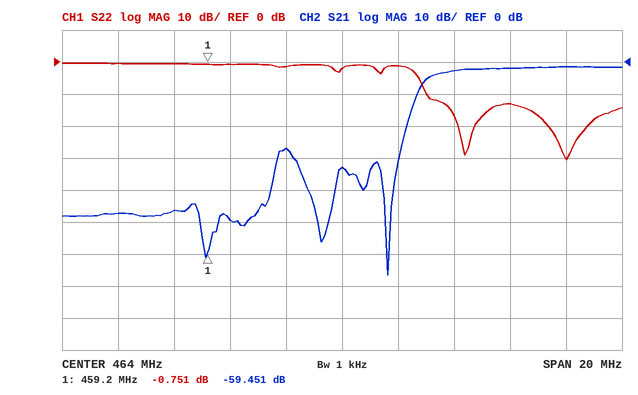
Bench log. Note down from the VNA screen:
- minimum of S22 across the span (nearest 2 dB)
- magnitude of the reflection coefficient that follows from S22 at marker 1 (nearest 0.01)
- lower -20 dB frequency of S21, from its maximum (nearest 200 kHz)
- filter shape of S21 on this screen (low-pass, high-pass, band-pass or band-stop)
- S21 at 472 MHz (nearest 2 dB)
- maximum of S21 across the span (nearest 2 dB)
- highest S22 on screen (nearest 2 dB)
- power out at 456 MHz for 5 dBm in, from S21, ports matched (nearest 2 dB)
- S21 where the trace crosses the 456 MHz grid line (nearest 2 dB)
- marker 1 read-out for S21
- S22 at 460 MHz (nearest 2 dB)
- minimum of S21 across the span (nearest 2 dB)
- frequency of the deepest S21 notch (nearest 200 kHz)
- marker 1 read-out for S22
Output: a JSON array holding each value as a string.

["-30 dB", "0.92", "466.2 MHz", "high-pass", "-2 dB", "-2 dB", "0 dB", "-42 dBm", "-48 dB", "-59.451 dB", "0 dB", "-66 dB", "465.6 MHz", "-0.751 dB"]
